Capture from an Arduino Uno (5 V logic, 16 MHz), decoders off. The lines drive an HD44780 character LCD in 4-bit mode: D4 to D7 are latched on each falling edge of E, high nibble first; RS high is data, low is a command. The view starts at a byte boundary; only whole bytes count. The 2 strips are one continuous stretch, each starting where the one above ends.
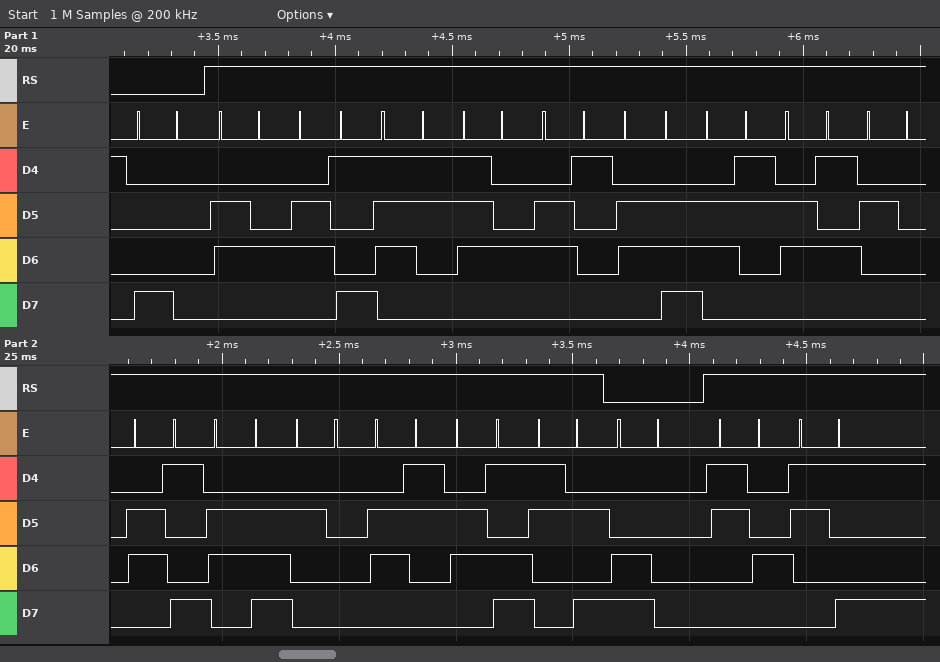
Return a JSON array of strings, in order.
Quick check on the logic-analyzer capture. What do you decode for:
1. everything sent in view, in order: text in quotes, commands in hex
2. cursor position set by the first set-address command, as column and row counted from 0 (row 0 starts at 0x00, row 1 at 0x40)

["0x80 \"distance in cm:\" 0xC0 \"49\"", "column 0, row 0"]
